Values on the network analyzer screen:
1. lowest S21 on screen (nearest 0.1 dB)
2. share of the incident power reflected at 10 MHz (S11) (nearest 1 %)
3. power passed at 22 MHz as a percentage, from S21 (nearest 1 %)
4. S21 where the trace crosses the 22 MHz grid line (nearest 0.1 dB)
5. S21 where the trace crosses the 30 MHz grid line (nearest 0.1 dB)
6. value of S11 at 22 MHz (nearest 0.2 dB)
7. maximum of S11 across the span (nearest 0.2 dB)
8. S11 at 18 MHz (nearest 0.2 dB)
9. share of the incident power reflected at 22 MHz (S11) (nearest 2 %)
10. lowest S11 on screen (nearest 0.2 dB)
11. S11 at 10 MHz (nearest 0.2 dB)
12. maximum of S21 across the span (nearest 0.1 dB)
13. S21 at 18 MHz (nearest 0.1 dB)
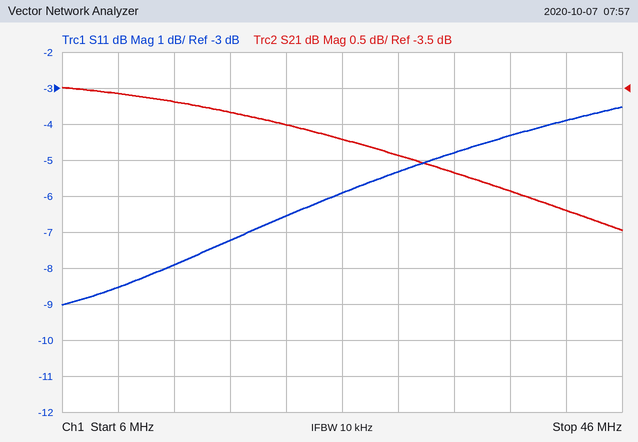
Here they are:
-5.5 dB
14 %
40 %
-4.0 dB
-4.4 dB
-6.6 dB
-3.6 dB
-7.2 dB
22 %
-9.0 dB
-8.6 dB
-3.5 dB
-3.8 dB
